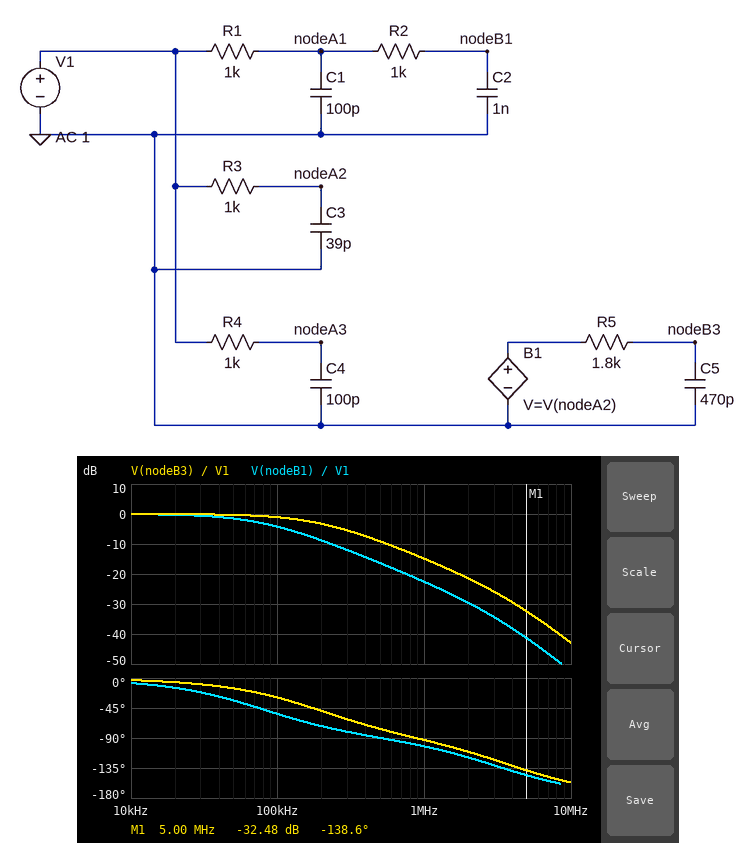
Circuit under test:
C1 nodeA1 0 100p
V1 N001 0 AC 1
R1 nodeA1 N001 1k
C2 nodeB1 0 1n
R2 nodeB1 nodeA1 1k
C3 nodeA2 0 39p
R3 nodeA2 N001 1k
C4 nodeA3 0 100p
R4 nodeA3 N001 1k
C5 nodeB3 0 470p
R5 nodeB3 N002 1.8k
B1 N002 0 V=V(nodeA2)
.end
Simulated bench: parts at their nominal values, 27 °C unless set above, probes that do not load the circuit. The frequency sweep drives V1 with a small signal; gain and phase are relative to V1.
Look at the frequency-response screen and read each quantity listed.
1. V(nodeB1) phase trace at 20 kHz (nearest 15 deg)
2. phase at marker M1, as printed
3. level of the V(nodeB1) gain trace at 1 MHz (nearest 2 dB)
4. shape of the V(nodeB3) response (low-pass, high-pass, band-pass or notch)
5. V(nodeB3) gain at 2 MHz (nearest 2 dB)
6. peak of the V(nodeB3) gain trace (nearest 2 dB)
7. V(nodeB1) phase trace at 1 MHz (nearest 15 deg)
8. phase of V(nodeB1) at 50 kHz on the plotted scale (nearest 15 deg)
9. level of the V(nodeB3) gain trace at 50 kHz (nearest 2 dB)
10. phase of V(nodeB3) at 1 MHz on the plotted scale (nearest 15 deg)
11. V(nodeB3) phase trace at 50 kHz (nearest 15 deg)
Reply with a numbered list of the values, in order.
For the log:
1. -15 deg
2. -138.6 deg
3. -22 dB
4. low-pass
5. -22 dB
6. 0 dB
7. -105 deg
8. -30 deg
9. 0 dB
10. -90 deg
11. -15 deg
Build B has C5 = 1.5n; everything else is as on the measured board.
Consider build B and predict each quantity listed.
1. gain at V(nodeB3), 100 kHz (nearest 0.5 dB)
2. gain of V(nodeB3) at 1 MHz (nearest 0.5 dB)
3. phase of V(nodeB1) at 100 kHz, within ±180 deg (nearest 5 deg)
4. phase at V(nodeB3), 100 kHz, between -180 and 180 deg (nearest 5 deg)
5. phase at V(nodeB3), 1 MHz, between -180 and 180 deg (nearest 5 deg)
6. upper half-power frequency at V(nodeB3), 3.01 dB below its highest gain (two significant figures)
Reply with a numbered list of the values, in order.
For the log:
1. -6.0 dB
2. -25.0 dB
3. -55 deg
4. -60 deg
5. -100 deg
6. 59 kHz
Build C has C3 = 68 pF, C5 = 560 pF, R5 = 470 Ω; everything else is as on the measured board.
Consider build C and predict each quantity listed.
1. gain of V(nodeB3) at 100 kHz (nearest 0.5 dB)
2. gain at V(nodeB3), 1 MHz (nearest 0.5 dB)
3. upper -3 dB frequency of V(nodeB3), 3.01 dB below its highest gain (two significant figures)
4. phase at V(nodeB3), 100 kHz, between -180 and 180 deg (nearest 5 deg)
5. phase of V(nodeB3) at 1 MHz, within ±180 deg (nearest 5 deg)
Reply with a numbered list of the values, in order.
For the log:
1. 0 dB
2. -6.5 dB
3. 570 kHz
4. -10 deg
5. -80 deg
